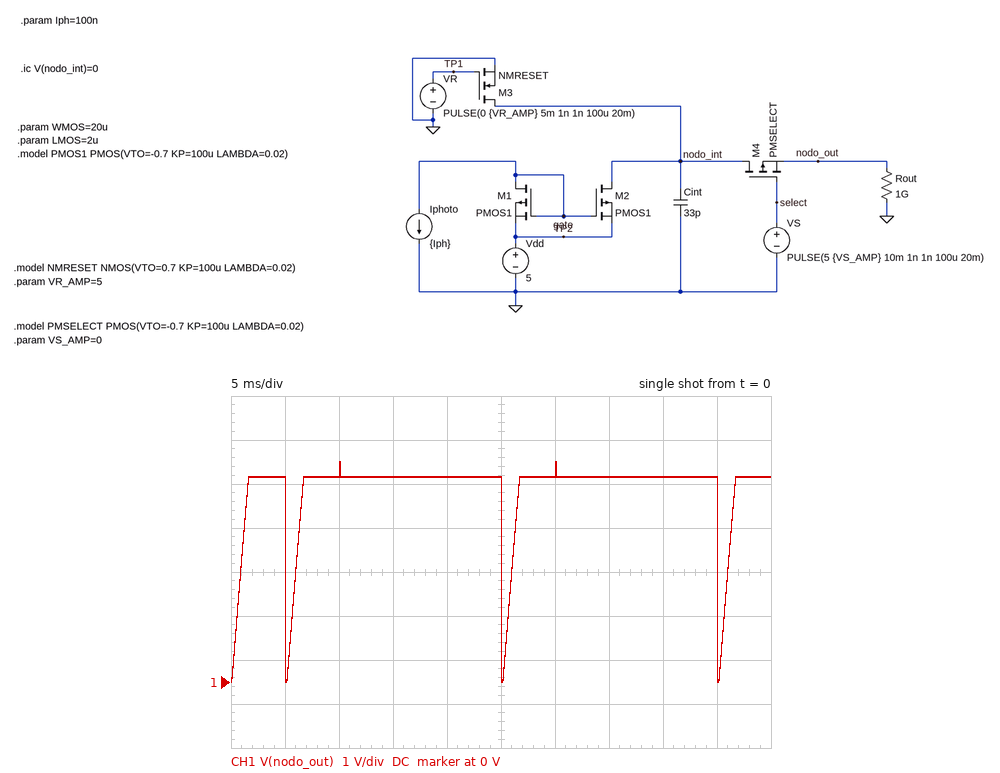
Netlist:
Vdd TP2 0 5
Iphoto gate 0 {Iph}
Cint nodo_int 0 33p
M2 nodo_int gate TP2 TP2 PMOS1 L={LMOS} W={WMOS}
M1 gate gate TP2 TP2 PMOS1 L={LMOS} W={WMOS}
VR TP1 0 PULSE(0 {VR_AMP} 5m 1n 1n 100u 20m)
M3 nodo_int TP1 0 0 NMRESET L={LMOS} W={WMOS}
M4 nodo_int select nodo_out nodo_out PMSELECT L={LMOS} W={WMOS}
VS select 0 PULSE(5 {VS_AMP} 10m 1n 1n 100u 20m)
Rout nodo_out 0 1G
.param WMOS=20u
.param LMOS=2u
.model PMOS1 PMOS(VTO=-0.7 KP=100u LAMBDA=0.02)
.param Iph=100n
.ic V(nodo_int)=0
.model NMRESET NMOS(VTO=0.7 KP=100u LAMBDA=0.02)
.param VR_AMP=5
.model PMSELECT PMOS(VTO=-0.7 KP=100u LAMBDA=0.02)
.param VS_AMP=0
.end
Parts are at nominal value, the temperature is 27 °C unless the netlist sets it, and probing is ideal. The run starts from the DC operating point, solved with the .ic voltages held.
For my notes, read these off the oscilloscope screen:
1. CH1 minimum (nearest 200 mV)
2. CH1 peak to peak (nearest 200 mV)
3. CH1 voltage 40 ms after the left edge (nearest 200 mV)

0 V
5.0 V
4.6 V
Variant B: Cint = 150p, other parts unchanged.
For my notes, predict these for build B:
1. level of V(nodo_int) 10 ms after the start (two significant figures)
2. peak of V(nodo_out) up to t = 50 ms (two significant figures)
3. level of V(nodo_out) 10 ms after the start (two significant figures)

3.4 V
4.7 V
3.1 V
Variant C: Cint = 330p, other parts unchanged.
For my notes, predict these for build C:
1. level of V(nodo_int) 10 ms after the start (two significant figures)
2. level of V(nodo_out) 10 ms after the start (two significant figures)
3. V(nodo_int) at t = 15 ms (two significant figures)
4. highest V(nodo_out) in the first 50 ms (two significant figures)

1.6 V
1.3 V
3.1 V
4.7 V
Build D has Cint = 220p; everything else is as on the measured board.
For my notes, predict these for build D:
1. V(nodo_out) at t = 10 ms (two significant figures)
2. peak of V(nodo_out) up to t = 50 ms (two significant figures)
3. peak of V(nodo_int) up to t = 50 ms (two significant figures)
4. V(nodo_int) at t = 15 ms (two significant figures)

2.0 V
4.7 V
5.0 V
4.6 V
